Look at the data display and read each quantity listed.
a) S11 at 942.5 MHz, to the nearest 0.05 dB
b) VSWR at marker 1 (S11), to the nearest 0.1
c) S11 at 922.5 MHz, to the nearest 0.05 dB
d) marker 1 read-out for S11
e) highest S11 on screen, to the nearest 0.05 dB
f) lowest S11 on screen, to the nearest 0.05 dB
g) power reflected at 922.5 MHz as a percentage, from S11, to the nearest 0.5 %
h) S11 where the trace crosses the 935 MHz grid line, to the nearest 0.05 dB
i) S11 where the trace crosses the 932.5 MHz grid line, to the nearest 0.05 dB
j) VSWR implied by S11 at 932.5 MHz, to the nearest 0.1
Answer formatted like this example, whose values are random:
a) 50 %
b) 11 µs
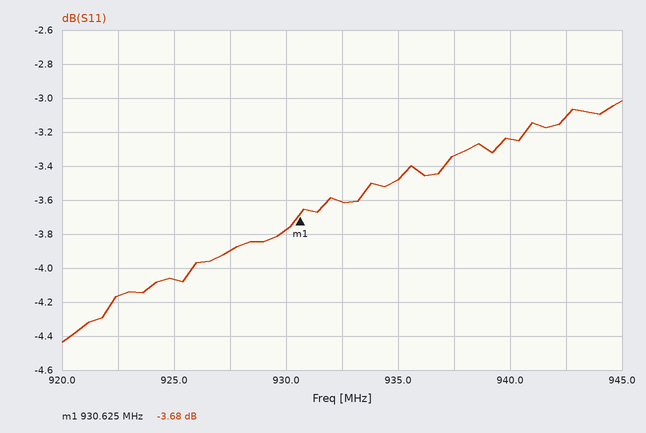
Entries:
a) -3.10 dB
b) 4.8
c) -4.15 dB
d) -3.68 dB
e) -3.00 dB
f) -4.45 dB
g) 38.5 %
h) -3.50 dB
i) -3.60 dB
j) 4.9
